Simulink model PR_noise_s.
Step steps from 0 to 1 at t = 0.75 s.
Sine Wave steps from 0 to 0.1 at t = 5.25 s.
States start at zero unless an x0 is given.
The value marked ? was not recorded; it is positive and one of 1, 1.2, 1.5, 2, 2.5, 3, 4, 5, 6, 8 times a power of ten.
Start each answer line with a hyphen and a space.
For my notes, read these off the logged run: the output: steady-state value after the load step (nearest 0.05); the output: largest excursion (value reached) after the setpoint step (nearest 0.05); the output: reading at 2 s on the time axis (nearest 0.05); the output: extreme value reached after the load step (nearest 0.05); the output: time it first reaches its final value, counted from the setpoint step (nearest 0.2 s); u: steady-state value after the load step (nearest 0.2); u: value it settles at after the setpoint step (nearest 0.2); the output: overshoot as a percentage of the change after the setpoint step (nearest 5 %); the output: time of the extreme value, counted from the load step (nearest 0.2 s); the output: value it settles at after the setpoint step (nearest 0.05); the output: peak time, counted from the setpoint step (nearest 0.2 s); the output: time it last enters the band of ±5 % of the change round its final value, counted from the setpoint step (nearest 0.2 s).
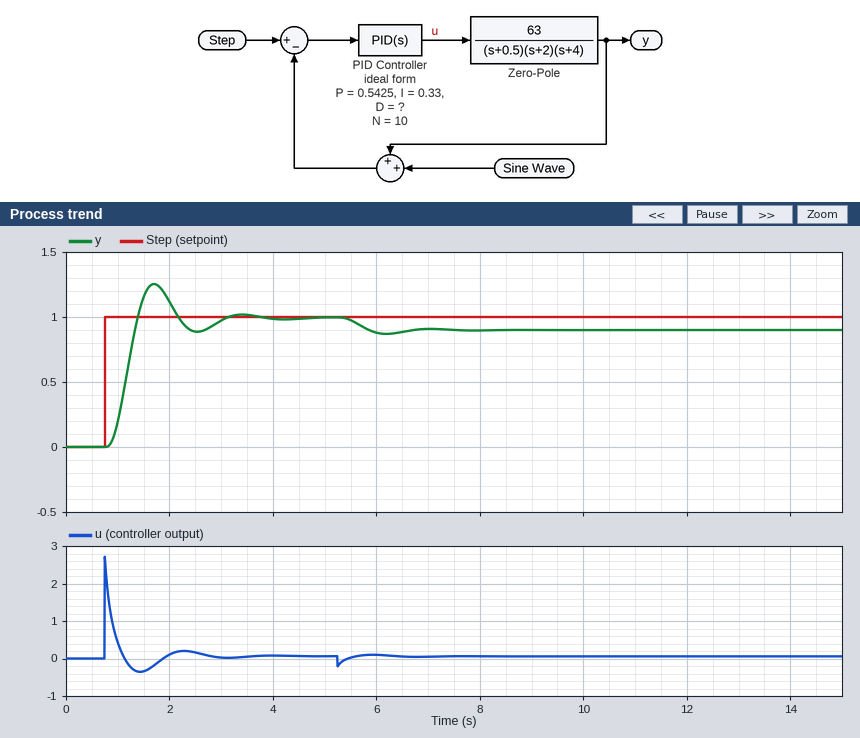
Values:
- 0.90
- 1.25
- 1.10
- 0.85
- 0.6 s
- 0.0
- 0.0
- 25 %
- 1.0 s
- 1.00
- 1.0 s
- 2.2 s
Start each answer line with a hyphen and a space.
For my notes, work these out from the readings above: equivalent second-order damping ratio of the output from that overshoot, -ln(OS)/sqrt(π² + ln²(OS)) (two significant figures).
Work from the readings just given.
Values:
- 0.40
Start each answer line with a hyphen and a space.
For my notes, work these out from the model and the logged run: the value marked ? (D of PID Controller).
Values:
- 0.4
